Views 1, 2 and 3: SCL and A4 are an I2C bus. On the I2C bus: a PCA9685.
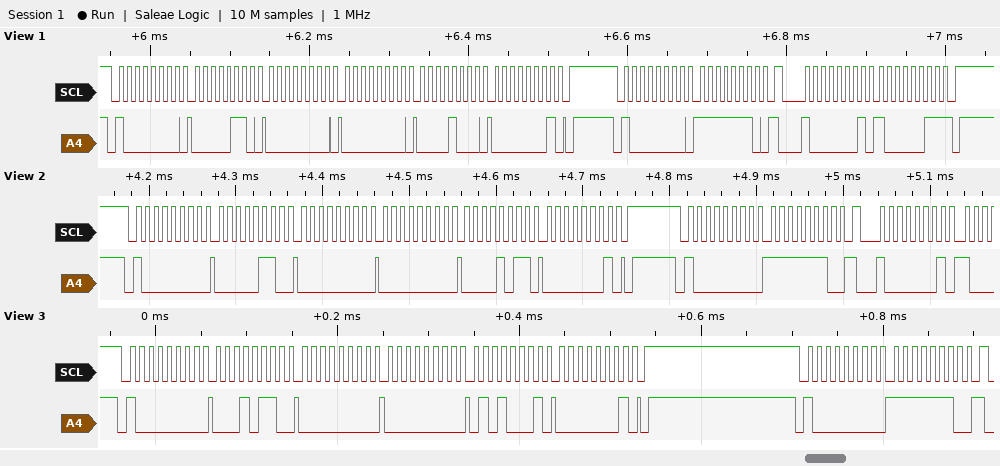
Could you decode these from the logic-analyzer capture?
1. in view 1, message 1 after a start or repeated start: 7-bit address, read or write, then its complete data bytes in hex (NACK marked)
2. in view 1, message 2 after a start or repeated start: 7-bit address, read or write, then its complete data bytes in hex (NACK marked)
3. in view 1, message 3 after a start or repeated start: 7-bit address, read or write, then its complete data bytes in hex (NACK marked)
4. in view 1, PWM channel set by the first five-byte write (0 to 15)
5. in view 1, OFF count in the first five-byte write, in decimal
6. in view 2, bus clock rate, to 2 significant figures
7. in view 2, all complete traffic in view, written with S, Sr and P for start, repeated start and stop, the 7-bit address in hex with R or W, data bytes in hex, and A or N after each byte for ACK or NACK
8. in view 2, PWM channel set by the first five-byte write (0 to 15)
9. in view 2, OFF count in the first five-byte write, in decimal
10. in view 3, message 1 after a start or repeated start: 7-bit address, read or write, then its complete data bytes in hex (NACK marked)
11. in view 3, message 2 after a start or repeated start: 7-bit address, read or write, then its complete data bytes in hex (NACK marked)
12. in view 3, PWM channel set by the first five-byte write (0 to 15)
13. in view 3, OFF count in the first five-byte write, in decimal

0x40 write: 06 00 00 08 01
0x40 write: FE
0x40 read: 83 NACK
0
264
100 kHz
S 40W A 06 A 00 A 00 A 0B A 01 A P S 40W A FE A Sr 40R A
0
267
0x40 write: 16 00 00 51 01
0x40 write: FE
4
337
